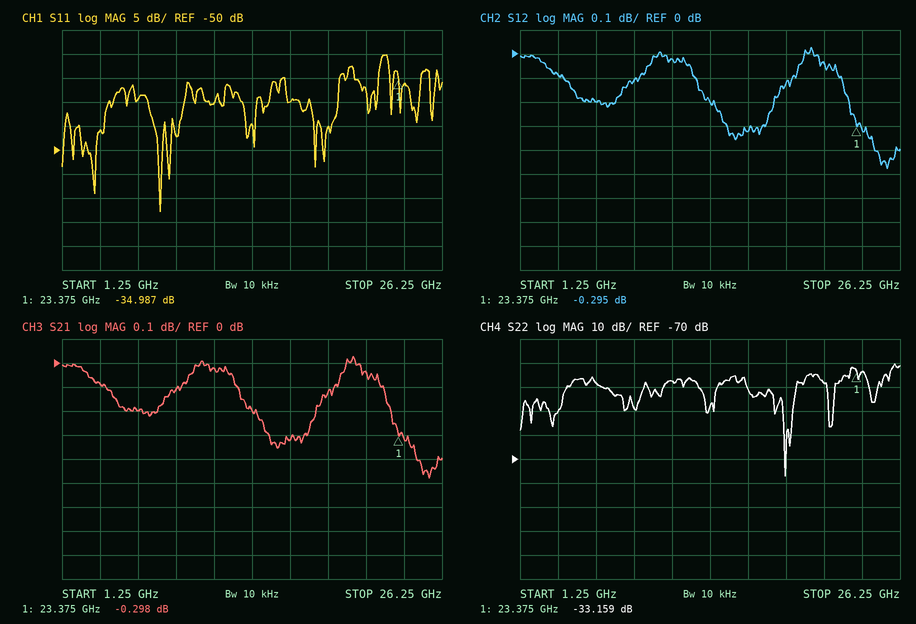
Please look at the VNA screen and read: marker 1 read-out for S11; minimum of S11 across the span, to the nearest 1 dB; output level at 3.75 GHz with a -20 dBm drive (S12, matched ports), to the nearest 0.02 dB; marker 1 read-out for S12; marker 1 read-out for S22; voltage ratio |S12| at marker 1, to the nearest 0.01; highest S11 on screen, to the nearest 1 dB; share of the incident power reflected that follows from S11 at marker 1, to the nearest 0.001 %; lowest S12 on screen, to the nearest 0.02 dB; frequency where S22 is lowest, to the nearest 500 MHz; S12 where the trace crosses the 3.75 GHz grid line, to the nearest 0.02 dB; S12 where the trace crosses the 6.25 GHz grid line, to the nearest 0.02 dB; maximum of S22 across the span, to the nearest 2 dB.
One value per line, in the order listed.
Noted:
-34.987 dB
-63 dB
-20.08 dBm
-0.295 dB
-33.159 dB
0.97
-30 dB
0.032 %
-0.48 dB
18.5 GHz
-0.08 dB
-0.20 dB
-30 dB
